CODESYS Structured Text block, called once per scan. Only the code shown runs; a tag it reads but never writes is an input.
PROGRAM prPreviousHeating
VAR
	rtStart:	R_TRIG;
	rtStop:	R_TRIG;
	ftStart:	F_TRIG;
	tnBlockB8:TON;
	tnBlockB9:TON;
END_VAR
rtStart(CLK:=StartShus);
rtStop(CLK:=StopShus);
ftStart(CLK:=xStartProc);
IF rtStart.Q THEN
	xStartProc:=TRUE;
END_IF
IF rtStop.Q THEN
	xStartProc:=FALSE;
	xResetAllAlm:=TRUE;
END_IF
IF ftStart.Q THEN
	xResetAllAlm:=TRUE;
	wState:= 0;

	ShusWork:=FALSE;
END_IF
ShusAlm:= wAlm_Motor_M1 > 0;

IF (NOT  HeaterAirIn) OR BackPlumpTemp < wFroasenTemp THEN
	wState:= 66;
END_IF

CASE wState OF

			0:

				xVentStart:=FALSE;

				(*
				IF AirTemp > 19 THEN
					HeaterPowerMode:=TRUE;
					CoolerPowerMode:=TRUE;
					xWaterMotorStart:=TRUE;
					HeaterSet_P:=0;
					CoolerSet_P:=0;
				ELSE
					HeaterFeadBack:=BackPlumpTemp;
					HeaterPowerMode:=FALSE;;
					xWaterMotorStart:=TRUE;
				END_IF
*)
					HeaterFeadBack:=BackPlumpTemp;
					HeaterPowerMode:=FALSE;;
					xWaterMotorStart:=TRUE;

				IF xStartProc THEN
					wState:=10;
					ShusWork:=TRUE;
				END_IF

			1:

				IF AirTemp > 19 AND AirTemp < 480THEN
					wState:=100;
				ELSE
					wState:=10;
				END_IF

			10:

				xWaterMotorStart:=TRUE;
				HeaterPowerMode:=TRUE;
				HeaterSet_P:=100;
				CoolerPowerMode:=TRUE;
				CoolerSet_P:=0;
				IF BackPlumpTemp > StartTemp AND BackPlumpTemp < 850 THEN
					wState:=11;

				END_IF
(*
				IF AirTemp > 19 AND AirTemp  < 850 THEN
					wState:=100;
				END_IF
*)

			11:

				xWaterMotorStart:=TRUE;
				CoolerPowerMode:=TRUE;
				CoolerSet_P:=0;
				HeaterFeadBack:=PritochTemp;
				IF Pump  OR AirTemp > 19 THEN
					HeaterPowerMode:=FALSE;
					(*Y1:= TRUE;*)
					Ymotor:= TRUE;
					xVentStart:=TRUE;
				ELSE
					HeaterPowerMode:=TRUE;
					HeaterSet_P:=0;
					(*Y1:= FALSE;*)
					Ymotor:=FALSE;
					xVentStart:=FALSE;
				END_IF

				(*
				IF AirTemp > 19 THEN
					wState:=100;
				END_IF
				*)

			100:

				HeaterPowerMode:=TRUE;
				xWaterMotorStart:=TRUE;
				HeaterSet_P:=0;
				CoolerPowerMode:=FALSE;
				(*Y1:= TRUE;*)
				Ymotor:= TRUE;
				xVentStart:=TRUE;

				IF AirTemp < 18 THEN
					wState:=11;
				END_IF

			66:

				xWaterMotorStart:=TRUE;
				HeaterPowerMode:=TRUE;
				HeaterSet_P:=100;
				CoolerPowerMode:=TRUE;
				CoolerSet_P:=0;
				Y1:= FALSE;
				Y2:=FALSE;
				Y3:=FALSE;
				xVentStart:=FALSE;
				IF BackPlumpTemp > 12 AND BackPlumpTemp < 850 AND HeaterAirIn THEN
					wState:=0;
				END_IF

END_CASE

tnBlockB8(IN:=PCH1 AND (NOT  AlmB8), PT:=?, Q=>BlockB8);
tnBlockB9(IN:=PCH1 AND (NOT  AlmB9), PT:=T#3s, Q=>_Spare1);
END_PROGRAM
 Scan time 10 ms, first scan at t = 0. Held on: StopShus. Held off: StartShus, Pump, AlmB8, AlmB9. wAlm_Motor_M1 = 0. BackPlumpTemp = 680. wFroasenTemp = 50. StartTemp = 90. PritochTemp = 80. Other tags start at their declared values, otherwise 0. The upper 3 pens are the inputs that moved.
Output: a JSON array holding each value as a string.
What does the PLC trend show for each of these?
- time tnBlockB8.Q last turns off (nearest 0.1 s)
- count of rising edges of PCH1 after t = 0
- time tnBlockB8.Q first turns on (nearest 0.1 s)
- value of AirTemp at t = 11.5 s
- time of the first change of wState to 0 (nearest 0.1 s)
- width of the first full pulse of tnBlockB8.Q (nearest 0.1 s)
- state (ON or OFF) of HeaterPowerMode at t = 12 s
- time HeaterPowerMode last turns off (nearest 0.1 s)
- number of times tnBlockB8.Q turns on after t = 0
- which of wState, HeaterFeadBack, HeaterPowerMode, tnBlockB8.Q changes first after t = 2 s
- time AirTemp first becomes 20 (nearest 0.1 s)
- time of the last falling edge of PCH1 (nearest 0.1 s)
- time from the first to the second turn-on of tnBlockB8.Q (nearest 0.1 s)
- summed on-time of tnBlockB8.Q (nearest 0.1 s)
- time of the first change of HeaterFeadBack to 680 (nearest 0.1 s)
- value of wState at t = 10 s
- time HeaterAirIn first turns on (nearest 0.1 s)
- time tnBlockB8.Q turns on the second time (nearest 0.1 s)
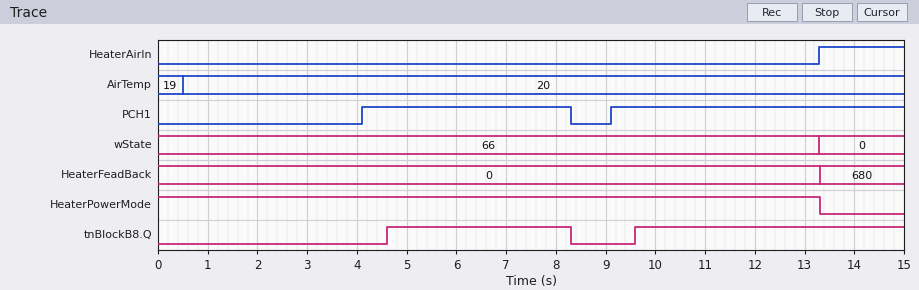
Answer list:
["8.3 s", "2", "4.6 s", "20", "13.3 s", "3.7 s", "ON", "13.3 s", "2", "tnBlockB8.Q", "0.5 s", "8.3 s", "5.0 s", "9.1 s", "13.3 s", "66", "13.3 s", "9.6 s"]
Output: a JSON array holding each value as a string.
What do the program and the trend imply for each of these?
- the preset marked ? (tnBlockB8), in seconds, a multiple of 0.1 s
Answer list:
["0.5 s"]
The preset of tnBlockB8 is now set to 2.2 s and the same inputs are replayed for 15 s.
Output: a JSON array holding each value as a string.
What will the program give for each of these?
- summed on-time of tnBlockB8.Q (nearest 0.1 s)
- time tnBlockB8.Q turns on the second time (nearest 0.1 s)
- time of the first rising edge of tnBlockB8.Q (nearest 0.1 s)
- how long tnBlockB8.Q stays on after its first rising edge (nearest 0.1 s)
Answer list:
["5.7 s", "11.3 s", "6.3 s", "2.0 s"]
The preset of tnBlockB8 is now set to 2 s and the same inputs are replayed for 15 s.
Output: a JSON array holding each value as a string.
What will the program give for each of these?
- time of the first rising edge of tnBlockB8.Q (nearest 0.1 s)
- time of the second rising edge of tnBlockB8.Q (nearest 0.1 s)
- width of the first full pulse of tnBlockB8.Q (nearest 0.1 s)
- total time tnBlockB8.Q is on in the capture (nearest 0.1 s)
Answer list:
["6.1 s", "11.1 s", "2.2 s", "6.1 s"]
